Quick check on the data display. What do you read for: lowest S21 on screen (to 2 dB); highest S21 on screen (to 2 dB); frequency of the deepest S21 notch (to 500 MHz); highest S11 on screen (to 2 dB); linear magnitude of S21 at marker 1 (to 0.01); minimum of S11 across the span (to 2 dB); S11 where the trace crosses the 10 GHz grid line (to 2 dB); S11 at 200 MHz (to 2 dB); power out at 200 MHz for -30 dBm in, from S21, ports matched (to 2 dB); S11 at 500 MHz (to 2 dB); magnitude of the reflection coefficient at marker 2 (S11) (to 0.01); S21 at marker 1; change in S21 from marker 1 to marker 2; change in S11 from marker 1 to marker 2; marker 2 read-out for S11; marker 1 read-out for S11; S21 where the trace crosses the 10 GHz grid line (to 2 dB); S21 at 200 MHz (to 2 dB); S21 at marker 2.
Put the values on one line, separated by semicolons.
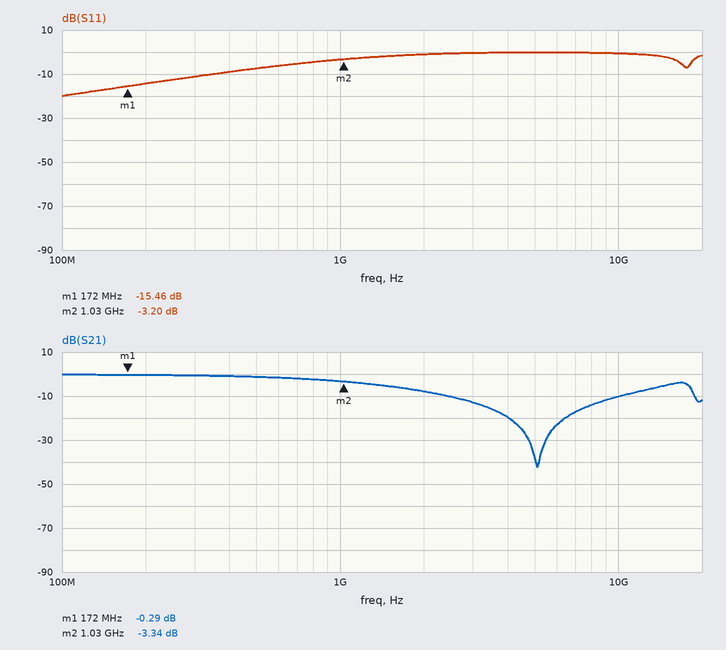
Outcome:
-42 dB; 0 dB; 5.0 GHz; 0 dB; 0.97; -20 dB; 0 dB; -14 dB; -30 dBm; -8 dB; 0.69; -0.29 dB; -3.05 dB; 12.26 dB; -3.20 dB; -15.46 dB; -10 dB; 0 dB; -3.34 dB
